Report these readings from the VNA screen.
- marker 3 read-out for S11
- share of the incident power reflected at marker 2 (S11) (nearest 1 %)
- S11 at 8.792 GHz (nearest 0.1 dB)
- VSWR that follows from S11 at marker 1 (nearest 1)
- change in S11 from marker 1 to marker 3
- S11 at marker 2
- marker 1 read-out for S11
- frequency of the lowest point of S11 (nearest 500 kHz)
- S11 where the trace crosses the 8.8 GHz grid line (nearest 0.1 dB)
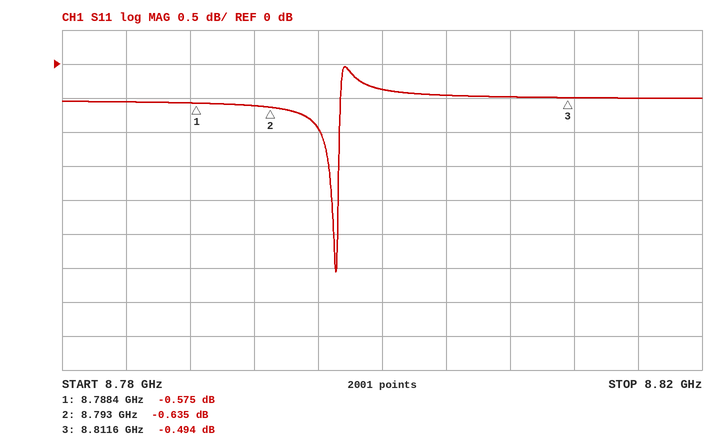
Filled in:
-0.494 dB
86 %
-0.6 dB
30
0.081 dB
-0.635 dB
-0.575 dB
8.7970 GHz
-0.4 dB
